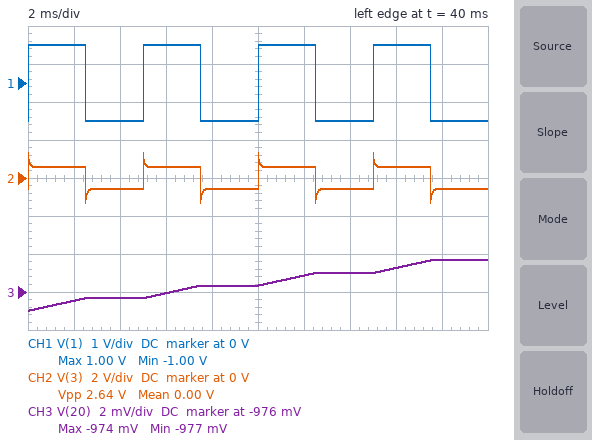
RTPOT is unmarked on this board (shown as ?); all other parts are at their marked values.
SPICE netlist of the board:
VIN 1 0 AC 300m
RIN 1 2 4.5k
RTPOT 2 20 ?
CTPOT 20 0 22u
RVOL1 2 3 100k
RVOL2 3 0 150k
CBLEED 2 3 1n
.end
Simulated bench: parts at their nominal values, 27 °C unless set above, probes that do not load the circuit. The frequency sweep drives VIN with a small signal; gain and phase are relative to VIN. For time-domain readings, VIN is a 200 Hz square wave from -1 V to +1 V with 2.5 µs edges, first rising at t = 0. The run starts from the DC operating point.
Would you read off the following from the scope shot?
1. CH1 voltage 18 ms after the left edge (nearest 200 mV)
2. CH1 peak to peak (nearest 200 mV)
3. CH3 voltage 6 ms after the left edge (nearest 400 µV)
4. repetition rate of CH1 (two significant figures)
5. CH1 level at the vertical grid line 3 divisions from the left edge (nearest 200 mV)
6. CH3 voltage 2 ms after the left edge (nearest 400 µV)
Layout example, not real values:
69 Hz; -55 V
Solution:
-1.0 V; 2.0 V; -976.0 mV; 200 Hz; 1.0 V; -976.4 mV
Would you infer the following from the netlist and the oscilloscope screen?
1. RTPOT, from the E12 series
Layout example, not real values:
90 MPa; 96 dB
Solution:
330 kΩ
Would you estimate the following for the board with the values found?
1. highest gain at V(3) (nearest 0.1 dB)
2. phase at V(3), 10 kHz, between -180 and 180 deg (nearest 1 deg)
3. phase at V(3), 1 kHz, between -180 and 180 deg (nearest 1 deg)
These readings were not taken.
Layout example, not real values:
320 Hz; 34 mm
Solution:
-0.4 dB; 6 deg; 11 deg
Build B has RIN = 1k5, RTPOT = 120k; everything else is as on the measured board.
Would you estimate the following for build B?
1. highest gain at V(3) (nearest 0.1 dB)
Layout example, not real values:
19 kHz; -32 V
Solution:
-0.2 dB
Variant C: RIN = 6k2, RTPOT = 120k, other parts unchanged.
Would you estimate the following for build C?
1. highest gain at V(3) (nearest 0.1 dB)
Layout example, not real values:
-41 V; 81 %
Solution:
-0.8 dB
